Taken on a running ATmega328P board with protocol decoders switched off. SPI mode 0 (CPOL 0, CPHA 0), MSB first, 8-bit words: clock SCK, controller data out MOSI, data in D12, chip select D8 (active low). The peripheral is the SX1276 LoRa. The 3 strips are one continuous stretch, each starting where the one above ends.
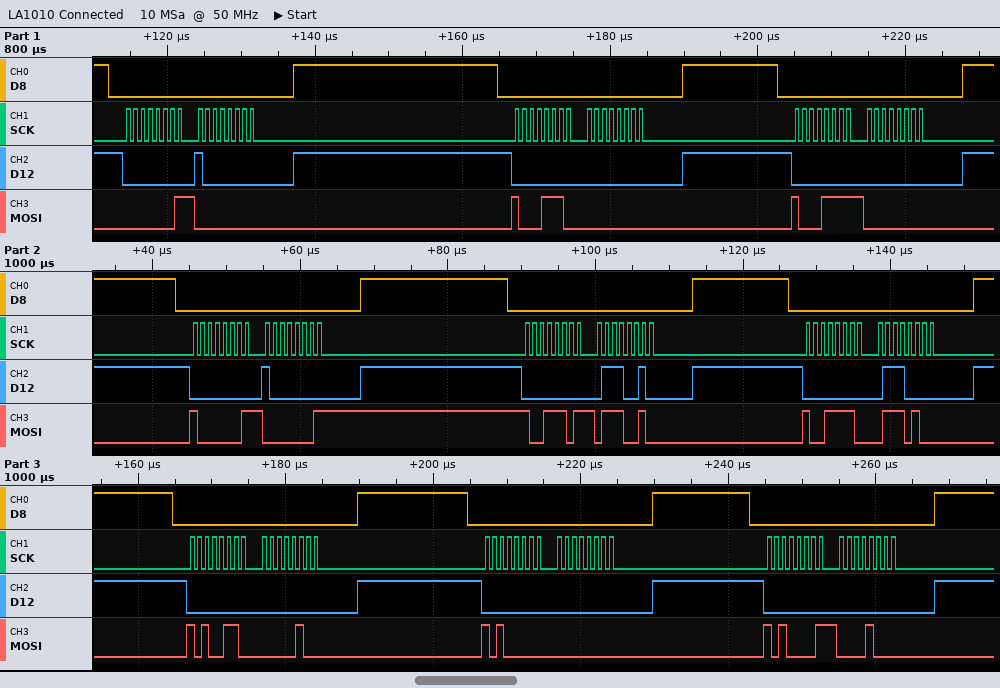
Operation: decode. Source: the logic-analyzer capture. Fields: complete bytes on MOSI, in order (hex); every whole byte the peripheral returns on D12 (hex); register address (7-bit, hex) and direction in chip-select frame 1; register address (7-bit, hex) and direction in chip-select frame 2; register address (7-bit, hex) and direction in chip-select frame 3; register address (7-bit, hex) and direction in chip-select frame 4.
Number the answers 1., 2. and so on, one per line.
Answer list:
1. 01 00 8E 00 8F 00 81 01 9D 72 9E 74 A6 04 A0 00 A1 08
2. 00 80 00 00 00 00 00 80 00 72 00 70 00 00 00 00 00 00
3. 0x01 read
4. 0x0E write
5. 0x0F write
6. 0x01 write
